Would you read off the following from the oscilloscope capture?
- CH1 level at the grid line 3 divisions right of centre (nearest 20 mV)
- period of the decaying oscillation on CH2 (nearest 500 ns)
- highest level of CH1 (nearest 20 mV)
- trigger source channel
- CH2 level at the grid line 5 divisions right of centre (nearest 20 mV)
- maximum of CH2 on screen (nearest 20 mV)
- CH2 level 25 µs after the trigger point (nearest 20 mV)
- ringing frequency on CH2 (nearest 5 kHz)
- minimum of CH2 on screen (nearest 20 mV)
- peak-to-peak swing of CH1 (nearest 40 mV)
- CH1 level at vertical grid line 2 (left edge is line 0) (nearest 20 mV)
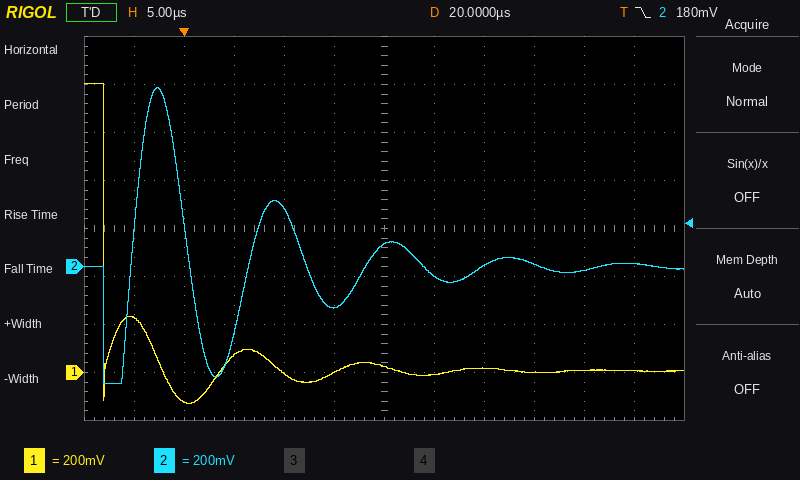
0 mV
11.5 µs
1.20 V
CH2
20 mV
740 mV
-40 mV
85 kHz
-480 mV
1.32 V
-120 mV
